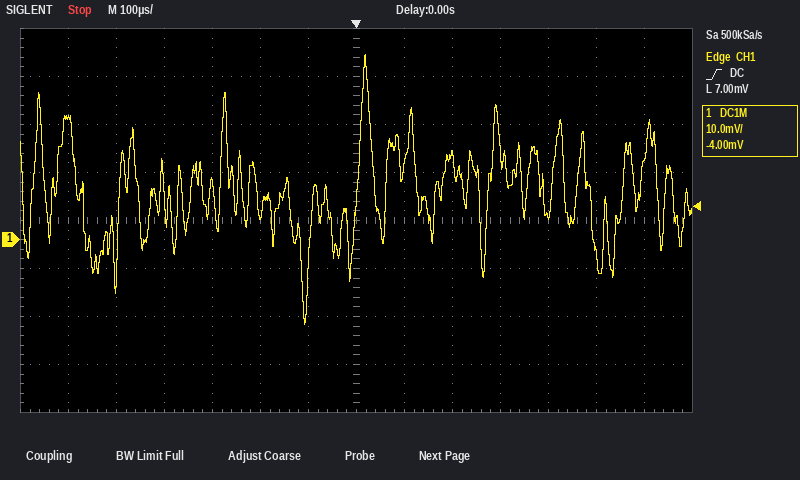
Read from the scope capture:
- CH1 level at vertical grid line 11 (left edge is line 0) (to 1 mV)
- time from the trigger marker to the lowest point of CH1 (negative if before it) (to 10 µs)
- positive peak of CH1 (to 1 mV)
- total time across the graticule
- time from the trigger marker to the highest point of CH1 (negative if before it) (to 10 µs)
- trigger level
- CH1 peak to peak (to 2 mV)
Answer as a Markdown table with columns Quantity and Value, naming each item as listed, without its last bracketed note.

| Quantity | Value |
|---|---|
| CH1 level at vertical grid line 11 (left edge is line 0) | 5 mV |
| time from the trigger marker to the lowest point of CH1 (negative if before it) | -110 µs |
| positive peak of CH1 | 39 mV |
| total time across the graticule | 1.4 ms |
| time from the trigger marker to the highest point of CH1 (negative if before it) | +20 µs |
| trigger level | 7.00 mV |
| CH1 peak to peak | 56 mV |
